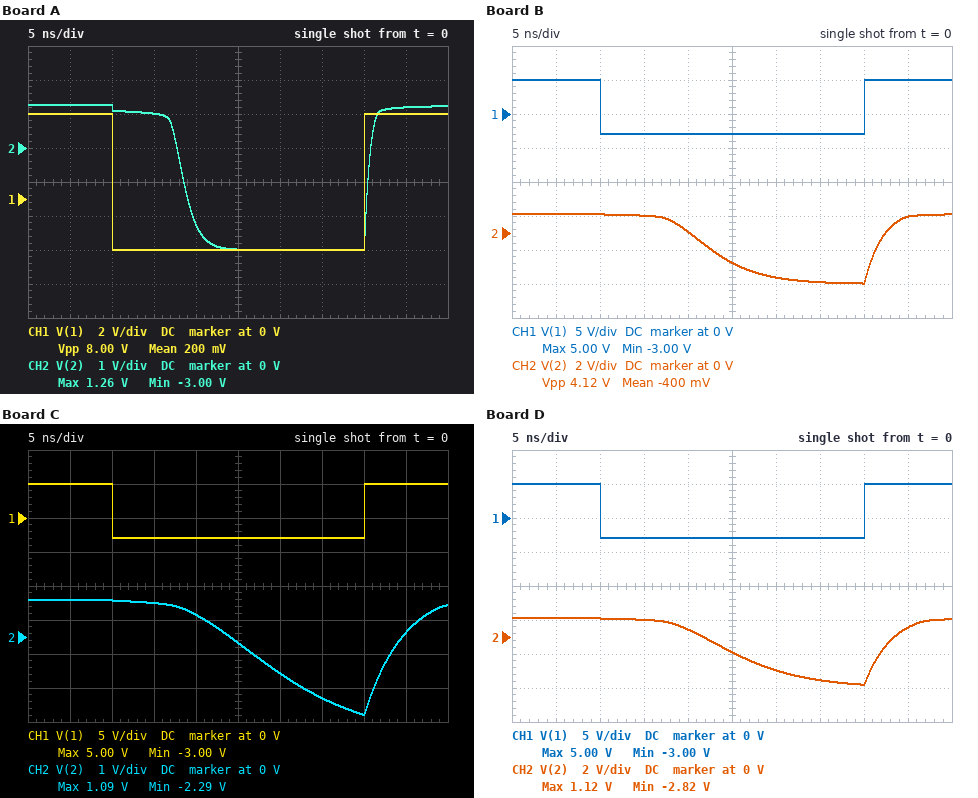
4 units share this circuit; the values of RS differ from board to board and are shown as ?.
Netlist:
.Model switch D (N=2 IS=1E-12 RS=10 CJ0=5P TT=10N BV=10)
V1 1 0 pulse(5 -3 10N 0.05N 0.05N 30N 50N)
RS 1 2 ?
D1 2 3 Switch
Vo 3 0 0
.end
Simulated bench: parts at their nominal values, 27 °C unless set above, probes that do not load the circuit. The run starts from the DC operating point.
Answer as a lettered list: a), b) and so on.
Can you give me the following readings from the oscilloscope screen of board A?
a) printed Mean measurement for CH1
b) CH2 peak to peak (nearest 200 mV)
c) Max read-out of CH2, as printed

a) 200 mV
b) 4.2 V
c) 1.26 V
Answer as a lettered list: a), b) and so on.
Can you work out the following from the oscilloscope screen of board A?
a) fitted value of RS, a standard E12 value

a) 470 Ω
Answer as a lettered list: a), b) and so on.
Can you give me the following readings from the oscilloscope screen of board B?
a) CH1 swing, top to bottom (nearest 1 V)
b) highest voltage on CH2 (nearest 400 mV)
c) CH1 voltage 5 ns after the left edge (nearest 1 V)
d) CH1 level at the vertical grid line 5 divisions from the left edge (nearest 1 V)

a) 8 V
b) 1.2 V
c) 5 V
d) -3 V
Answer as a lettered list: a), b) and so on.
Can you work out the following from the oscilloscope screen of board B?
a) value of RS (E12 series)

a) 1.5 kΩ
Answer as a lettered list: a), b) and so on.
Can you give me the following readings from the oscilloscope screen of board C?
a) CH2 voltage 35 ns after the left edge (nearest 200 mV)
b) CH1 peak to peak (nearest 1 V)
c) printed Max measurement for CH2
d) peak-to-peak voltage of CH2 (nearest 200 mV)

a) -1.8 V
b) 8 V
c) 1.09 V
d) 3.4 V
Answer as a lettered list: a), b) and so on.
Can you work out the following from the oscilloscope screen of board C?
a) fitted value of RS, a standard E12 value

a) 3.3 kΩ
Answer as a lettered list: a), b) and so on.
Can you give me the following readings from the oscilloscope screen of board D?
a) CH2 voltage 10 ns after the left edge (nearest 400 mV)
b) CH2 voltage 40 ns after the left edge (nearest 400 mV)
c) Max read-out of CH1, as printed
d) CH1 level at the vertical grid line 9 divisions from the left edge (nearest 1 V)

a) 1.2 V
b) -2.8 V
c) 5.00 V
d) 5 V
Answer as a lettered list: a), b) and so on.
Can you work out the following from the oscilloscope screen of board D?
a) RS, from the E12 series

a) 2.2 kΩ
